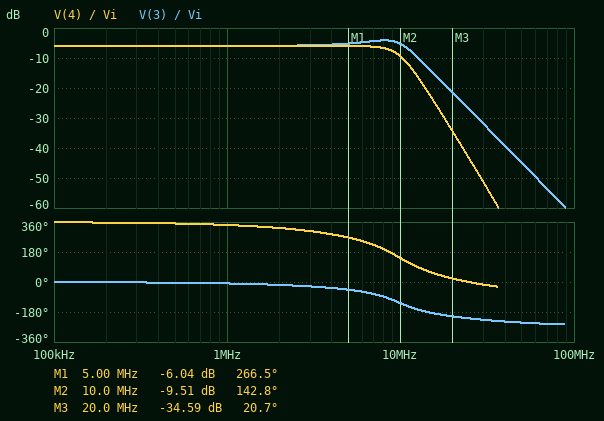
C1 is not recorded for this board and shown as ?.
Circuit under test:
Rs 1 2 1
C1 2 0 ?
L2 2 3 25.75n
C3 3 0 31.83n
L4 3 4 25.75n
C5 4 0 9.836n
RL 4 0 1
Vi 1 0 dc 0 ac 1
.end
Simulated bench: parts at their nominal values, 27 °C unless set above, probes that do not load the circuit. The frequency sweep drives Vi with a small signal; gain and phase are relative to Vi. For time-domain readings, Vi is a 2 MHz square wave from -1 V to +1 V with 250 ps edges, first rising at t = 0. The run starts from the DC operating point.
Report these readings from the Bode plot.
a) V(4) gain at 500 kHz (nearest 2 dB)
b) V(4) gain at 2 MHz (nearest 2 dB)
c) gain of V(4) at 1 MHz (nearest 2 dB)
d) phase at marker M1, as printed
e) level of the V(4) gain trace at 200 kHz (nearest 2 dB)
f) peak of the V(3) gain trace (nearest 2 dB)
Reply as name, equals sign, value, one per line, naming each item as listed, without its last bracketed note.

V(4) gain at 500 kHz = -6 dB
V(4) gain at 2 MHz = -6 dB
gain of V(4) at 1 MHz = -6 dB
phase at marker M1, as printed = 266.5 deg
level of the V(4) gain trace at 200 kHz = -6 dB
peak of the V(3) gain trace = -4 dB
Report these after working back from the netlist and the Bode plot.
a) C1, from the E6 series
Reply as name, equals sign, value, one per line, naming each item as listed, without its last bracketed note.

C1, from the E6 series = 6.8 nF
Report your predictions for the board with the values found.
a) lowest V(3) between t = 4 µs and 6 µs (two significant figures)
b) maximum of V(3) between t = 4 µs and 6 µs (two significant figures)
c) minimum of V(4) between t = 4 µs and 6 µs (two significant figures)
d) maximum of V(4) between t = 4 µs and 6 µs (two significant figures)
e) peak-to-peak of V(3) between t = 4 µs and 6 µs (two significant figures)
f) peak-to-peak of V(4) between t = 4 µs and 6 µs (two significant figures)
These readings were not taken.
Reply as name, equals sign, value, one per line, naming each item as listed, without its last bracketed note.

lowest V(3) between t = 4 µs and 6 µs = -700 mV
maximum of V(3) between t = 4 µs and 6 µs = 700 mV
minimum of V(4) between t = 4 µs and 6 µs = -620 mV
maximum of V(4) between t = 4 µs and 6 µs = 620 mV
peak-to-peak of V(3) between t = 4 µs and 6 µs = 1.4 V
peak-to-peak of V(4) between t = 4 µs and 6 µs = 1.2 V
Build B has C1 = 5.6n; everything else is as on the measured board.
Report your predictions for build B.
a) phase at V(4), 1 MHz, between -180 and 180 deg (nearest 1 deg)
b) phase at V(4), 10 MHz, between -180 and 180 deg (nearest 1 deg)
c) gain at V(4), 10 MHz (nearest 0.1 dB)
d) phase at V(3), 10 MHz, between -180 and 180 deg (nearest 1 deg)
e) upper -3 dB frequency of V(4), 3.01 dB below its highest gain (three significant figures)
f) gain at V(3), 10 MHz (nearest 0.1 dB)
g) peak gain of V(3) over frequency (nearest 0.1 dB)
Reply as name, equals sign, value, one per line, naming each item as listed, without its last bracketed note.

phase at V(4), 1 MHz, between -180 and 180 deg = -18 deg
phase at V(4), 10 MHz, between -180 and 180 deg = 146 deg
gain at V(4), 10 MHz = -9.7 dB
phase at V(3), 10 MHz, between -180 and 180 deg = -124 deg
upper -3 dB frequency of V(4), 3.01 dB below its highest gain = 9.66 MHz
gain at V(3), 10 MHz = -5.6 dB
peak gain of V(3) over frequency = -4.2 dB
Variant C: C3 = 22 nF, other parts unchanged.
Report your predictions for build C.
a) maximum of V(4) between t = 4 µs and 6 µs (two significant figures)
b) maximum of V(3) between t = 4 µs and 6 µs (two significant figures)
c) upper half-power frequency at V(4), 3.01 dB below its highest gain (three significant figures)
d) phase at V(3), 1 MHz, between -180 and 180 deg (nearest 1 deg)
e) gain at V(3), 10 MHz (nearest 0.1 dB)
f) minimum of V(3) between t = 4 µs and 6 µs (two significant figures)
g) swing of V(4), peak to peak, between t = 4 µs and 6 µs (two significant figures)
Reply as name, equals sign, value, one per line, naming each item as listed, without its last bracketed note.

maximum of V(4) between t = 4 µs and 6 µs = 630 mV
maximum of V(3) between t = 4 µs and 6 µs = 780 mV
upper half-power frequency at V(4), 3.01 dB below its highest gain = 11.8 MHz
phase at V(3), 1 MHz, between -180 and 180 deg = -7 deg
gain at V(3), 10 MHz = -2.2 dB
minimum of V(3) between t = 4 µs and 6 µs = -780 mV
swing of V(4), peak to peak, between t = 4 µs and 6 µs = 1.3 V
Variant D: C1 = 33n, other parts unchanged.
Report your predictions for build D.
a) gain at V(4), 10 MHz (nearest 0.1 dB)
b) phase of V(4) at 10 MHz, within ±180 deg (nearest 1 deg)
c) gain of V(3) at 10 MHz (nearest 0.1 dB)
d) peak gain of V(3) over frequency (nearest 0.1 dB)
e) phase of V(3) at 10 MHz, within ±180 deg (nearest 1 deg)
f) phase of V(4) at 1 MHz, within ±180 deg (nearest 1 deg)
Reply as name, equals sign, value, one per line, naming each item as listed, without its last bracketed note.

gain at V(4), 10 MHz = -11.1 dB
phase of V(4) at 10 MHz, within ±180 deg = 75 deg
gain of V(3) at 10 MHz = -6.9 dB
peak gain of V(3) over frequency = -3.6 dB
phase of V(3) at 10 MHz, within ±180 deg = 165 deg
phase of V(4) at 1 MHz, within ±180 deg = -23 deg
